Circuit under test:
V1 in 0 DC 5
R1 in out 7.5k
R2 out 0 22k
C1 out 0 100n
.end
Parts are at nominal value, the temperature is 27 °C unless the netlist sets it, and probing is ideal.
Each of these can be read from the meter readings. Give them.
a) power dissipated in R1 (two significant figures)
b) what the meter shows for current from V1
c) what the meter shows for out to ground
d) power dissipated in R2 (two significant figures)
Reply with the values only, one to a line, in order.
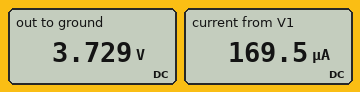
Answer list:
220 µW
169.5 µA
3.729 V
630 µW
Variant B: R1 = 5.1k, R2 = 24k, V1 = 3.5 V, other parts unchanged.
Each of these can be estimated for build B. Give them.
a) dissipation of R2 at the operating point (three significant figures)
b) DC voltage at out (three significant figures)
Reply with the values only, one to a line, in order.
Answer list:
347 µW
2.89 V
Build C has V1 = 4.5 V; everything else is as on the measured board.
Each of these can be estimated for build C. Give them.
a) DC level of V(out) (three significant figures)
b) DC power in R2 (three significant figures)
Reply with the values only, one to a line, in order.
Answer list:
3.36 V
512 µW
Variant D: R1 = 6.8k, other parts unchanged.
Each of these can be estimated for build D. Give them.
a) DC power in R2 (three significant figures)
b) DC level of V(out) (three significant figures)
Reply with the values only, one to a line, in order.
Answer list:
663 µW
3.82 V
